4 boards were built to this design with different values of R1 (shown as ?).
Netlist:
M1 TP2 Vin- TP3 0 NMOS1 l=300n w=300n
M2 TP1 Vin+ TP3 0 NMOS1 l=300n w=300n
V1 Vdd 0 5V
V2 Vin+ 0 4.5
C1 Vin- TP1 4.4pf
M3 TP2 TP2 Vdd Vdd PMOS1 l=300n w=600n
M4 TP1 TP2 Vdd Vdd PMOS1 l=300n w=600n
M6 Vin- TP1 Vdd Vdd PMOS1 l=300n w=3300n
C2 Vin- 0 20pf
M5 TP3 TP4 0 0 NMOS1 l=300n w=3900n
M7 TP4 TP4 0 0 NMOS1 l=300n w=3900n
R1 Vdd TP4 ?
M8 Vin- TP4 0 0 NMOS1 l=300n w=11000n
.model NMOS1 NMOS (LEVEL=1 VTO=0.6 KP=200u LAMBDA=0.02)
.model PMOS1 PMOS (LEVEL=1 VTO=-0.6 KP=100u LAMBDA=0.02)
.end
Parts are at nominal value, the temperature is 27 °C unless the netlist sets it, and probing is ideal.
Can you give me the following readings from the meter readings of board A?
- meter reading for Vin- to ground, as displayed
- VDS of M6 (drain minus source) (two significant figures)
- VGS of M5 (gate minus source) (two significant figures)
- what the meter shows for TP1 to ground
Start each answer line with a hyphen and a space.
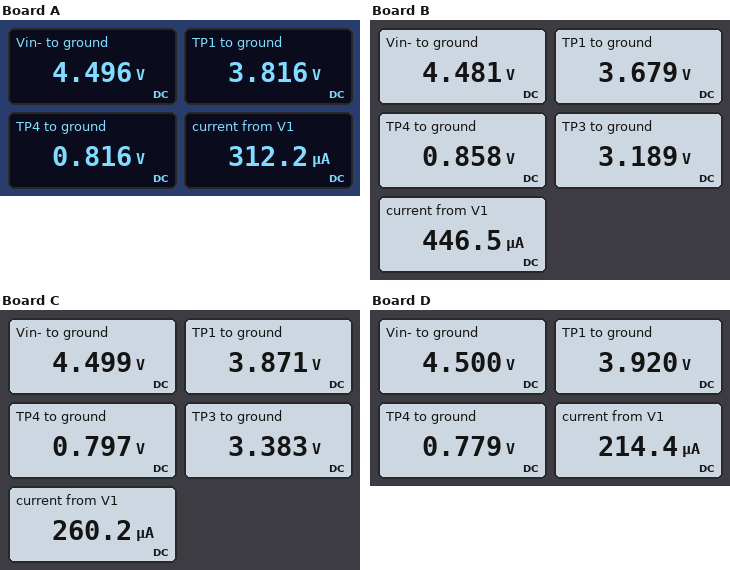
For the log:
- 4.496 V
- -500 mV
- 820 mV
- 3.816 V
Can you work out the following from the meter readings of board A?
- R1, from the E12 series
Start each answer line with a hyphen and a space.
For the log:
- 68 kΩ
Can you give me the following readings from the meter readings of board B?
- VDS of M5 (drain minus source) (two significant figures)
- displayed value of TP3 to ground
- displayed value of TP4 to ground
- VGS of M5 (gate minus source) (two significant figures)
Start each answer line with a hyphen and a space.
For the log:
- 3.2 V
- 3.189 V
- 0.858 V
- 860 mV
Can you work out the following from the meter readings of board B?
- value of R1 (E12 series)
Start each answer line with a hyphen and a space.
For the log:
- 47 kΩ
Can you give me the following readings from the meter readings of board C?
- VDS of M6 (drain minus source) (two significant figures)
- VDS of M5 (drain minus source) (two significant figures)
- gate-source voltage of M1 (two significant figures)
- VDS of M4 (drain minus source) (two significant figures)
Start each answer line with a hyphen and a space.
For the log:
- -500 mV
- 3.4 V
- 1.1 V
- -1.1 V
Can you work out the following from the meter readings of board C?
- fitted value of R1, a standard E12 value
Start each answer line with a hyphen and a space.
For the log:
- 82 kΩ
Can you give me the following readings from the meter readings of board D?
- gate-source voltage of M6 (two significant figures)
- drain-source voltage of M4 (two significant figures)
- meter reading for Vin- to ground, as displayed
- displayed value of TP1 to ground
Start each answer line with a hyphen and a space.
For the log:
- -1.1 V
- -1.1 V
- 4.500 V
- 3.920 V
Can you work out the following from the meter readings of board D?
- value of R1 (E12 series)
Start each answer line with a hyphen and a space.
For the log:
- 100 kΩ
